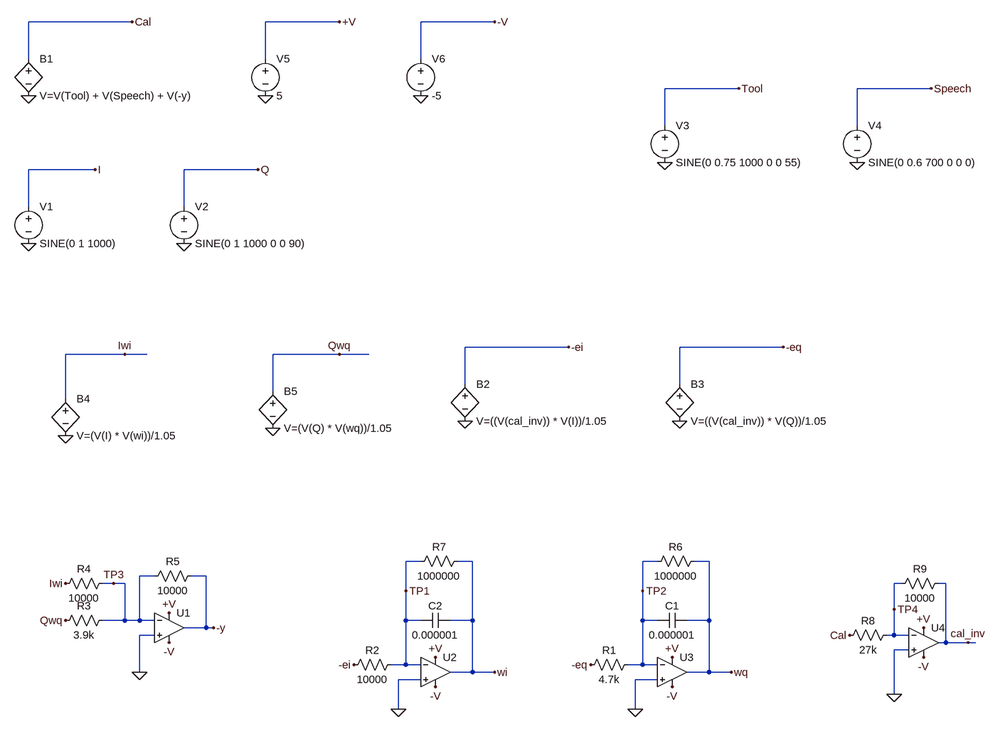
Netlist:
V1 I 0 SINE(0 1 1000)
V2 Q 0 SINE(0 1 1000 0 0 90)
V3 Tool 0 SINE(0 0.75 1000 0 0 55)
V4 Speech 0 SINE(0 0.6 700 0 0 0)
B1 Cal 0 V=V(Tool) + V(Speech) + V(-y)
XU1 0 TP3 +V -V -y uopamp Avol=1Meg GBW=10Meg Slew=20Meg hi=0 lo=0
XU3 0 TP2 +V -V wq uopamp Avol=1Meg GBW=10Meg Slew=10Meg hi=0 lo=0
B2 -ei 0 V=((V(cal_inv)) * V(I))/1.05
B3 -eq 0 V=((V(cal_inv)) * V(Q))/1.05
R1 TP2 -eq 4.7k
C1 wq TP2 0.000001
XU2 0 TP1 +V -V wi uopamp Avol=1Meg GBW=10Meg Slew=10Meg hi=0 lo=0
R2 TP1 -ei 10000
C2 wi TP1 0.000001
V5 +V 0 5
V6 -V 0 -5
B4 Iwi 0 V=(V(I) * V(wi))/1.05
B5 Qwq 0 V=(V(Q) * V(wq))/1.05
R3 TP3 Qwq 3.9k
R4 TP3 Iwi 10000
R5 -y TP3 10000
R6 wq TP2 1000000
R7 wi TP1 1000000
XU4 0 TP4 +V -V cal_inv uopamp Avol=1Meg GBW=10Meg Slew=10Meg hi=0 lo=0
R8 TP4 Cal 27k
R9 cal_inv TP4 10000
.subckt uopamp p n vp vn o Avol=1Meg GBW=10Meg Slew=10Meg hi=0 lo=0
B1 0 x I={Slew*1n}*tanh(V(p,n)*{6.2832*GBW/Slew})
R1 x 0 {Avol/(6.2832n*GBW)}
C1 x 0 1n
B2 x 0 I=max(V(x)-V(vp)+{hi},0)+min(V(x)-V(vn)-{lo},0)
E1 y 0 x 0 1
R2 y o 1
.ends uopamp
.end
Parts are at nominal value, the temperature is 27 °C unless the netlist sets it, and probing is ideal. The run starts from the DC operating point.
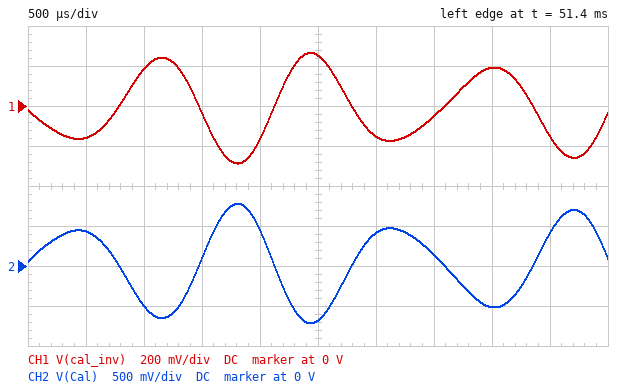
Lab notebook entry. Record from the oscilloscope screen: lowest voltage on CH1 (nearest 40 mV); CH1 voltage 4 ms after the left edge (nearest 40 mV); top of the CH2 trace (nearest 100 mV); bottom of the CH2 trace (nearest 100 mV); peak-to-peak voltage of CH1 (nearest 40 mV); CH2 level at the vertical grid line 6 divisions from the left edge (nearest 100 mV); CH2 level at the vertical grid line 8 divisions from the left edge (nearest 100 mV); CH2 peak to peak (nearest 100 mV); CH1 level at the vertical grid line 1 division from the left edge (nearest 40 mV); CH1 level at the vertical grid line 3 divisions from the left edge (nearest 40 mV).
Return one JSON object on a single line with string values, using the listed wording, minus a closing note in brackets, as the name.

{"lowest voltage on CH1": "-280 mV", "CH1 voltage 4 ms after the left edge": "200 mV", "top of the CH2 trace": "800 mV", "bottom of the CH2 trace": "-700 mV", "peak-to-peak voltage of CH1": "560 mV", "CH2 level at the vertical grid line 6 divisions from the left edge": "400 mV", "CH2 level at the vertical grid line 8 divisions from the left edge": "-500 mV", "CH2 peak to peak": "1.5 V", "CH1 level at the vertical grid line 1 division from the left edge": "-160 mV", "CH1 level at the vertical grid line 3 divisions from the left edge": "-40 mV"}
